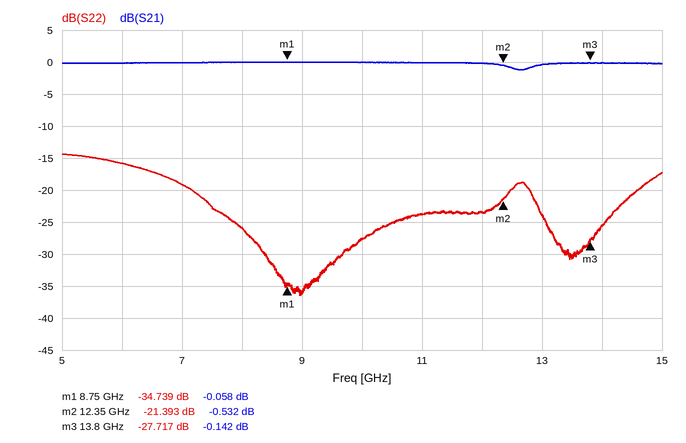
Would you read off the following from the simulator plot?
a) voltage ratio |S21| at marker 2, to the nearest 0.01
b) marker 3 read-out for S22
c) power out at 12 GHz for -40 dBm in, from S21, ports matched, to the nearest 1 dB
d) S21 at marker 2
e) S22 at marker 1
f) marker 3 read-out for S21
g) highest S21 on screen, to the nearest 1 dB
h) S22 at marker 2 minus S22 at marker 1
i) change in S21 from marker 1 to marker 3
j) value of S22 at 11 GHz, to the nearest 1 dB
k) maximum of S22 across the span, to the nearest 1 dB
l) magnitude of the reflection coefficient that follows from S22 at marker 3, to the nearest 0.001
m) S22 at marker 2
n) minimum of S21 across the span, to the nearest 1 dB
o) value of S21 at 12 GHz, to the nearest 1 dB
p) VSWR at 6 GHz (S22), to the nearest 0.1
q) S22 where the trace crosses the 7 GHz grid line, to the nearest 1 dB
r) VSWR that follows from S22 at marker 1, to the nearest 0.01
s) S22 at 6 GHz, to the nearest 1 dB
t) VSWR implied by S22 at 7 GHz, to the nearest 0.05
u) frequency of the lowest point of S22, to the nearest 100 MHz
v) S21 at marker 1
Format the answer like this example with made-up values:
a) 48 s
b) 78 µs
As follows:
a) 0.94
b) -27.717 dB
c) -40 dBm
d) -0.532 dB
e) -34.739 dB
f) -0.142 dB
g) 0 dB
h) 13.346 dB
i) -0.084 dB
j) -24 dB
k) -14 dB
l) 0.041
m) -21.393 dB
n) -1 dB
o) 0 dB
p) 1.4
q) -19 dB
r) 1.04
s) -16 dB
t) 1.25
u) 9.0 GHz
v) -0.058 dB
